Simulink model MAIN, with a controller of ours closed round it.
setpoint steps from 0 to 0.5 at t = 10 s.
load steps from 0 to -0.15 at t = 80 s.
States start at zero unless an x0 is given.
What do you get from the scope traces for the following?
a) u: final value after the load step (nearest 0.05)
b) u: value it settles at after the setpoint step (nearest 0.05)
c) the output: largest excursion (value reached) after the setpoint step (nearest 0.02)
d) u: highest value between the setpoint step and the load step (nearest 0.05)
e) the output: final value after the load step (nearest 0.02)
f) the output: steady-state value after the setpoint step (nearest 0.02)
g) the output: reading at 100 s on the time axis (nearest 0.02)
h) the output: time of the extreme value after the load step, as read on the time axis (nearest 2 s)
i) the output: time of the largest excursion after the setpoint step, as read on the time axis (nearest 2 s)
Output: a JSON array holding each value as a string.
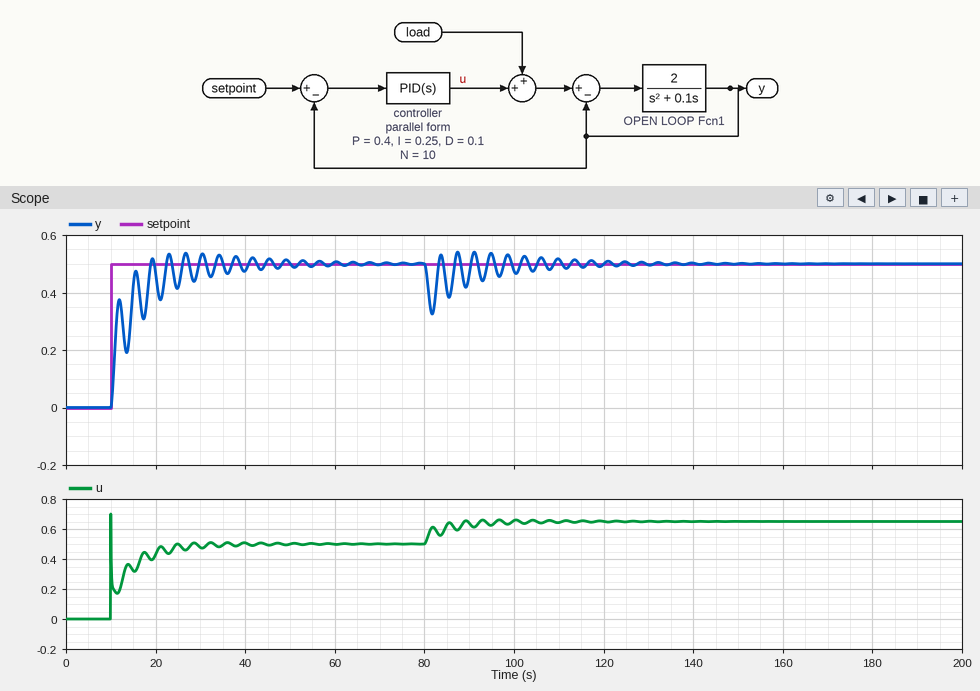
["0.65", "0.50", "0.54", "0.70", "0.50", "0.50", "0.48", "82 s", "26 s"]
